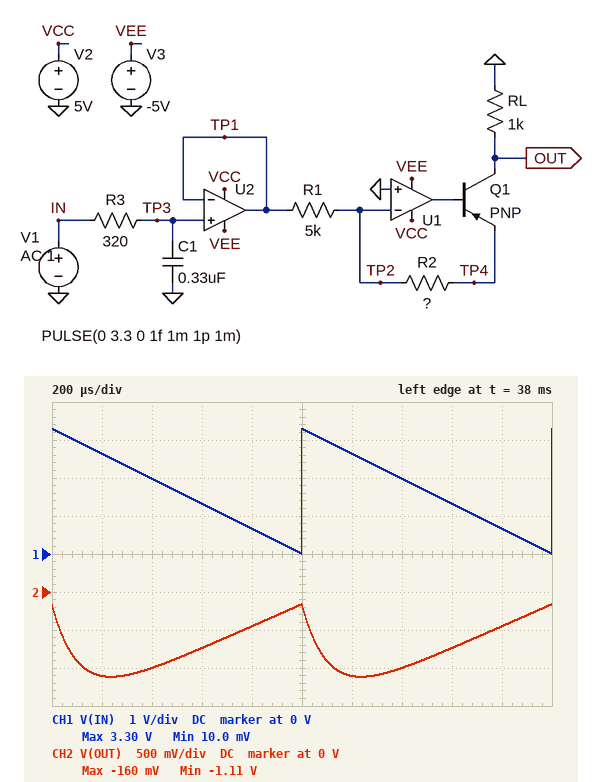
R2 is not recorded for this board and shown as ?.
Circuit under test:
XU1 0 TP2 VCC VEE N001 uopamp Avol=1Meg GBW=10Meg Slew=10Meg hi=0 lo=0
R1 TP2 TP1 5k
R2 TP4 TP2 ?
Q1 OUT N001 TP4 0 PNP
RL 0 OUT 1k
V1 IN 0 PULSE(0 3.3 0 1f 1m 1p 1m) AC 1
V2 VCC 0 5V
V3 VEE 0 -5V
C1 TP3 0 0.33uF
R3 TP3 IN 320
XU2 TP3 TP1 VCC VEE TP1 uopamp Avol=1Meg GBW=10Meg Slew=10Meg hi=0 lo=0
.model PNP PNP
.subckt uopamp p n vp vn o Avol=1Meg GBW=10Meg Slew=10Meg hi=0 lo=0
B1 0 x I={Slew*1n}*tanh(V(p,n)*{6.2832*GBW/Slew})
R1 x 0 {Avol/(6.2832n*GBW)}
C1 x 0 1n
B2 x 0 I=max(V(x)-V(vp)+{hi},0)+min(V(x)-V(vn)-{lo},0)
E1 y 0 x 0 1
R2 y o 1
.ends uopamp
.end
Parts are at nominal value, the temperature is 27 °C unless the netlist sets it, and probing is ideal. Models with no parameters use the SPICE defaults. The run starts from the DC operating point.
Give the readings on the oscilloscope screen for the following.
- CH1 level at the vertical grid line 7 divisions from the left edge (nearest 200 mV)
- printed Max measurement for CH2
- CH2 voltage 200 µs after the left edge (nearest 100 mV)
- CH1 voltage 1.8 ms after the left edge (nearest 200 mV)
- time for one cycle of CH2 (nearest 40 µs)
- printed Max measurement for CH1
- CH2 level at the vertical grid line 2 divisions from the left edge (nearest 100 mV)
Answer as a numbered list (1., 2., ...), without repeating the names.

1. 2.0 V
2. -160 mV
3. -1.1 V
4. 600 mV
5. 1.00 ms
6. 3.30 V
7. -1.0 V
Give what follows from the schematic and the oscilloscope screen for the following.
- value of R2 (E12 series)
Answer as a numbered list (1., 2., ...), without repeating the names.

1. 2.2 kΩ
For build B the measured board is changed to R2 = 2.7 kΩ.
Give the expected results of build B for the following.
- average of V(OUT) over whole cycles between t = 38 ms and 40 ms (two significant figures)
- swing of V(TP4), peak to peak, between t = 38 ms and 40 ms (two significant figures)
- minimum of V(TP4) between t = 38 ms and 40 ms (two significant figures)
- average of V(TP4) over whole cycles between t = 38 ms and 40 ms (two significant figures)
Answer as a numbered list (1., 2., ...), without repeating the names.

1. -900 mV
2. 1.2 V
3. -1.4 V
4. -890 mV
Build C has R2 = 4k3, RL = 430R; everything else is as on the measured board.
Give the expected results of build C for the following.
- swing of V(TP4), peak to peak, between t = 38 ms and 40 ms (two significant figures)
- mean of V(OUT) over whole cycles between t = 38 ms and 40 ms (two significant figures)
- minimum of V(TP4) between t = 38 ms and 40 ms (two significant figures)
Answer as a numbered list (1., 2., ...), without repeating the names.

1. 1.9 V
2. -1.4 V
3. -2.2 V
